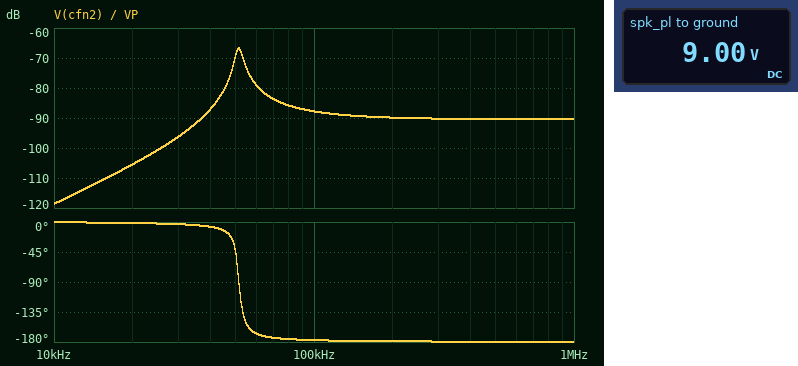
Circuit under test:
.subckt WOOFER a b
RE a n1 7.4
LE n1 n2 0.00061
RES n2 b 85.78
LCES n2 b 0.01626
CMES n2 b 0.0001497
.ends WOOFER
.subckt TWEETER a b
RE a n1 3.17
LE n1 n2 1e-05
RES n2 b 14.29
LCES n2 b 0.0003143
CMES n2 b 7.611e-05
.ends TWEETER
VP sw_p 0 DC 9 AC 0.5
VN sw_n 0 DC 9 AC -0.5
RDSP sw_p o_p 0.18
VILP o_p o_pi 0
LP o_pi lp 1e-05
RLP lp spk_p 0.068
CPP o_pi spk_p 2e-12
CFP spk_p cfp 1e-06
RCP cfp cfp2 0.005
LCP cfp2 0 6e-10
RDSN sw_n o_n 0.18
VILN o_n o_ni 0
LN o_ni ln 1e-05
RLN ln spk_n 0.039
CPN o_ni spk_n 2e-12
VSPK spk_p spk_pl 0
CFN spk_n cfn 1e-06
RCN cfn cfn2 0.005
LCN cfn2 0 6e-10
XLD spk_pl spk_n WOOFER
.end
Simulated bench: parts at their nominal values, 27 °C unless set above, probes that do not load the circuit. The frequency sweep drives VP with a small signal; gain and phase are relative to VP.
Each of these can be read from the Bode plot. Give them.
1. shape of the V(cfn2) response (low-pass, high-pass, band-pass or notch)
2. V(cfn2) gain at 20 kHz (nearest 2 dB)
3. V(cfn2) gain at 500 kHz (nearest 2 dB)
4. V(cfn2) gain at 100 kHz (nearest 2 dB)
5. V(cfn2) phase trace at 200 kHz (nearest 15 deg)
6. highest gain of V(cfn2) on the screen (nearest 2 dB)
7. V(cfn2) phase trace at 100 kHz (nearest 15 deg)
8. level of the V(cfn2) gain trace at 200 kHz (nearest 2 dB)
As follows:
high-pass
-106 dB
-90 dB
-88 dB
-180 deg
-66 dB
-180 deg
-90 dB
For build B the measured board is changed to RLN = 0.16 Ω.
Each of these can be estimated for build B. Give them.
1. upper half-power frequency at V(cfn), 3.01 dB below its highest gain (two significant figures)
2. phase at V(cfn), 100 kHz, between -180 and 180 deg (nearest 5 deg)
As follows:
54 kHz
100 deg
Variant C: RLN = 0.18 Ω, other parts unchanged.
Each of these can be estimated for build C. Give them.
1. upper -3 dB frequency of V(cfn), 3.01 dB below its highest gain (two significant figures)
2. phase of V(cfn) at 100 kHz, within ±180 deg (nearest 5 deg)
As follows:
54 kHz
100 deg
